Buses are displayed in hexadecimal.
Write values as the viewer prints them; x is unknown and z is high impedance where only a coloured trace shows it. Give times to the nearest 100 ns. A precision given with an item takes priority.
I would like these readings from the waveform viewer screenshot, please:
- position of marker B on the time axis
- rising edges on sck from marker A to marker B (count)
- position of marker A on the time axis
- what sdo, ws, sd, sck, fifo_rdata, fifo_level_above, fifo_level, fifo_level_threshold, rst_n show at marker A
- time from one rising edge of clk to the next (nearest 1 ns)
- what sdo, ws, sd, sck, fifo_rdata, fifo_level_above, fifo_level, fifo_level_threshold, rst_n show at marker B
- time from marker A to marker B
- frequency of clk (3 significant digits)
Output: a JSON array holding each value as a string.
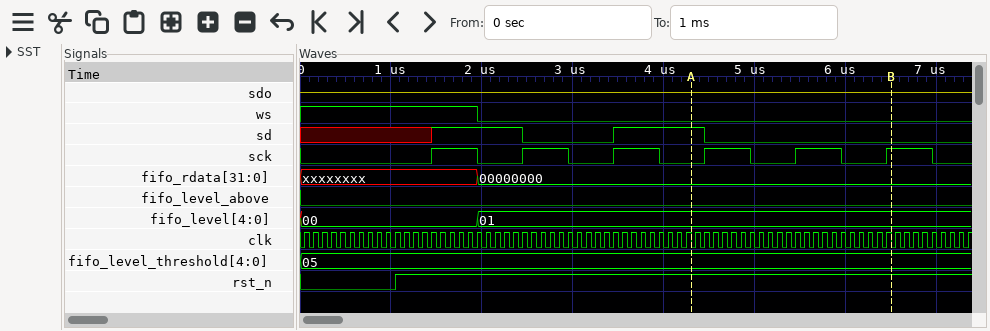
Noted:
["6500 ns", "3", "4300 ns", "sdo=z, ws=0, sd=1, sck=0, fifo_rdata=00000000, fifo_level_above=0, fifo_level=01, fifo_level_threshold=05, rst_n=1", "100 ns", "sdo=z, ws=0, sd=0, sck=1, fifo_rdata=00000000, fifo_level_above=0, fifo_level=01, fifo_level_threshold=05, rst_n=1", "2200 ns", "10.0 MHz"]
